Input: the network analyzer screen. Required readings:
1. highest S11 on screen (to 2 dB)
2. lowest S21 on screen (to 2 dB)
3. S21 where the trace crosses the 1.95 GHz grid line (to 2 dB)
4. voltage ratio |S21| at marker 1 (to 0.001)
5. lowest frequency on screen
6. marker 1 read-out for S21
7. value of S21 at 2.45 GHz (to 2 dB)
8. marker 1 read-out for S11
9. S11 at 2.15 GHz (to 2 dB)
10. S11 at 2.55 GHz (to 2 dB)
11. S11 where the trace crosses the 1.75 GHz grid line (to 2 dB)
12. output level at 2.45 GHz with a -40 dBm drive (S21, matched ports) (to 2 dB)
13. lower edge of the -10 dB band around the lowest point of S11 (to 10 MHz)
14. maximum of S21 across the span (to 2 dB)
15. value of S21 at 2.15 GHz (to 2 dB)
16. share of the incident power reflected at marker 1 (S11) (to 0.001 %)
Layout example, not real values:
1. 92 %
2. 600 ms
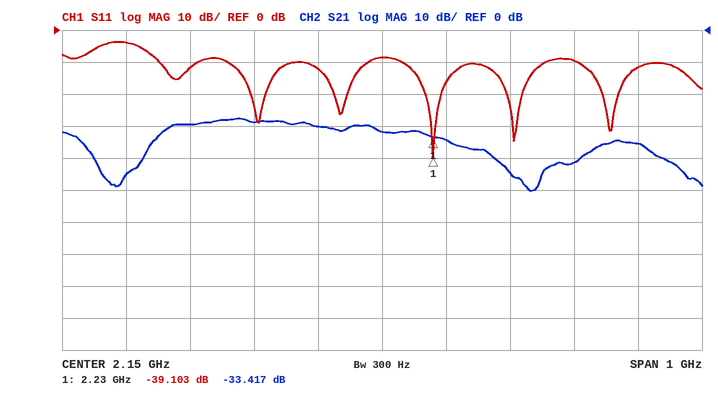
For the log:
1. -4 dB
2. -50 dB
3. -28 dB
4. 0.021
5. 1.65 GHz
6. -33.417 dB
7. -42 dB
8. -39.103 dB
9. -8 dB
10. -12 dB
11. -4 dB
12. -82 dBm
13. 2.18 GHz
14. -28 dB
15. -32 dB
16. 0.012 %
